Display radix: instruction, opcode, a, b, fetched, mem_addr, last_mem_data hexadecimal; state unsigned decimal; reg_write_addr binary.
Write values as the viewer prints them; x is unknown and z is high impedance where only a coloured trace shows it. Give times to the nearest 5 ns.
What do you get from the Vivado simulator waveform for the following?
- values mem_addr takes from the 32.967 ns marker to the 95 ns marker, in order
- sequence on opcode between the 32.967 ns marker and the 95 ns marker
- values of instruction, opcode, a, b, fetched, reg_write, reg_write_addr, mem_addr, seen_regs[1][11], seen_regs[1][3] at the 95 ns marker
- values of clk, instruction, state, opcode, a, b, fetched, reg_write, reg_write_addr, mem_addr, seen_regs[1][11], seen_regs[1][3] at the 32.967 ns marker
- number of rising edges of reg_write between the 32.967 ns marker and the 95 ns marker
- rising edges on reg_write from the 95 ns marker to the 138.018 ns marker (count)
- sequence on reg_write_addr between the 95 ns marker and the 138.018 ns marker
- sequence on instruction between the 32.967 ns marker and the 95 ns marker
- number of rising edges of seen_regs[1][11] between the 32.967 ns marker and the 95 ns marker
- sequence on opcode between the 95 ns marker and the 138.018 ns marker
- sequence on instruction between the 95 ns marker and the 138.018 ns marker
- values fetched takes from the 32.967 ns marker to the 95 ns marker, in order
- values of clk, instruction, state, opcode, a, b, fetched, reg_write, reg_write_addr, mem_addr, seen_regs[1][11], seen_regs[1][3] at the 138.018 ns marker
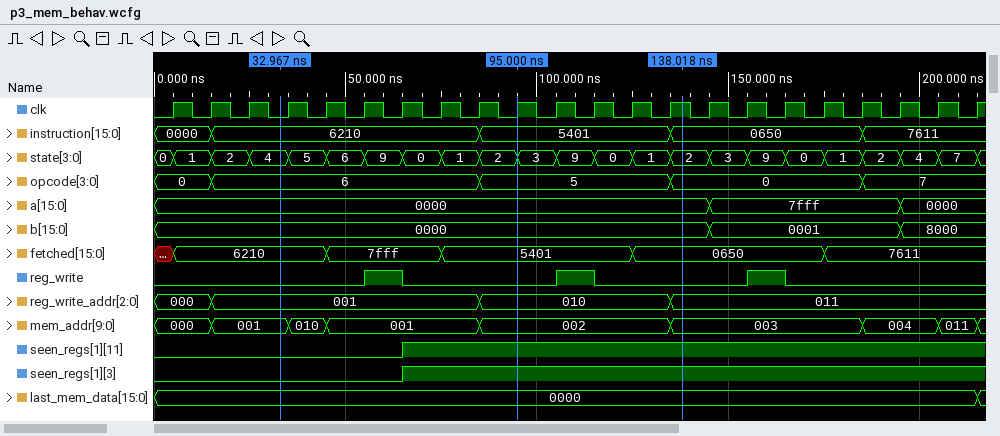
001, 010, 001, 002
6, 5
instruction=5401, opcode=5, a=0000, b=0000, fetched=5401, reg_write=0, reg_write_addr=010, mem_addr=002, seen_regs[1][11]=1, seen_regs[1][3]=1
clk=0, instruction=6210, state=4, opcode=6, a=0000, b=0000, fetched=6210, reg_write=0, reg_write_addr=001, mem_addr=001, seen_regs[1][11]=0, seen_regs[1][3]=0
1
1
010, 011
6210, 5401
1
5, 0
5401, 0650
6210, 7fff, 5401
clk=1, instruction=0650, state=2, opcode=0, a=0000, b=0000, fetched=0650, reg_write=0, reg_write_addr=011, mem_addr=003, seen_regs[1][11]=1, seen_regs[1][3]=1
